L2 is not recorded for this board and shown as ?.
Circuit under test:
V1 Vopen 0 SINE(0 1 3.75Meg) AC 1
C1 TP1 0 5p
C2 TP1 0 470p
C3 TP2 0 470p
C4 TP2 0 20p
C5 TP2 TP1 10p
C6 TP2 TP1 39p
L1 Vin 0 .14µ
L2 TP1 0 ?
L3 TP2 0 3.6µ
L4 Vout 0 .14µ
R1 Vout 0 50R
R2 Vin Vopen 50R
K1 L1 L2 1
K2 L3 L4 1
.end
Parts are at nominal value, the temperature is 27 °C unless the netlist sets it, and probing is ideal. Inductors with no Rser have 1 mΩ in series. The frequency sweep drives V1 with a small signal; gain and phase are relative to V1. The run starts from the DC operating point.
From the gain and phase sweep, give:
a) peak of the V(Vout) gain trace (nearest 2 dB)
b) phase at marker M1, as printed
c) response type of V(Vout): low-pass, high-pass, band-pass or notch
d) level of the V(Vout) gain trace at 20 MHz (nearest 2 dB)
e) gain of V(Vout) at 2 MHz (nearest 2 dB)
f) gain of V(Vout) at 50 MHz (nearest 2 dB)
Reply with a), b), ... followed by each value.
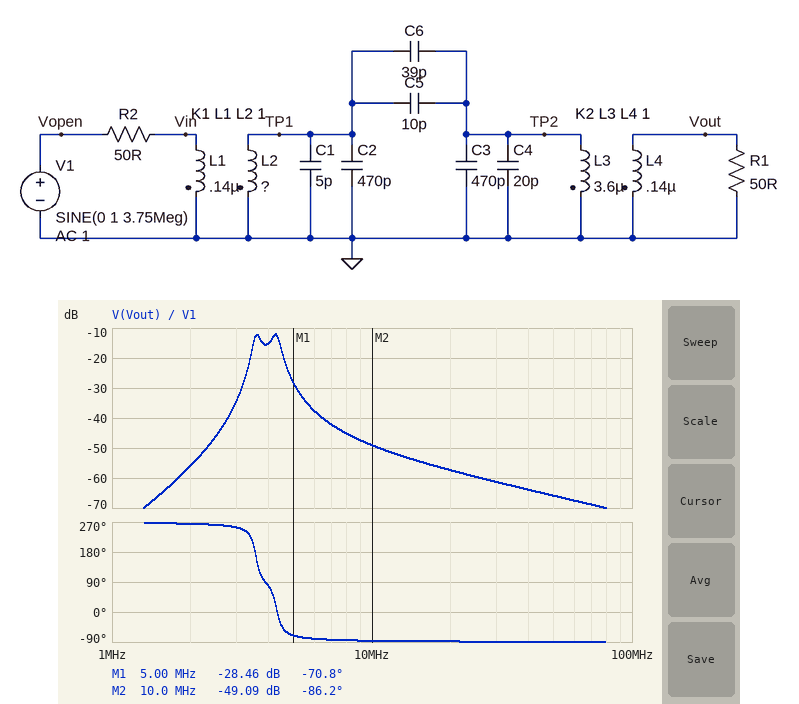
a) -12 dB
b) -70.8 deg
c) band-pass
d) -58 dB
e) -56 dB
f) -66 dB
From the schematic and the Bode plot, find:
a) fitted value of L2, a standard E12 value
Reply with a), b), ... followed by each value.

a) 2.7 µH
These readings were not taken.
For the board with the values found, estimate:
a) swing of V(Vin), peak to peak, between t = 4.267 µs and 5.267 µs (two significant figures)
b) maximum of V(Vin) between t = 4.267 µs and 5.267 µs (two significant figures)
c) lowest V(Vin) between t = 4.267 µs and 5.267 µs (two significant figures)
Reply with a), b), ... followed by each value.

a) 460 mV
b) 230 mV
c) -230 mV
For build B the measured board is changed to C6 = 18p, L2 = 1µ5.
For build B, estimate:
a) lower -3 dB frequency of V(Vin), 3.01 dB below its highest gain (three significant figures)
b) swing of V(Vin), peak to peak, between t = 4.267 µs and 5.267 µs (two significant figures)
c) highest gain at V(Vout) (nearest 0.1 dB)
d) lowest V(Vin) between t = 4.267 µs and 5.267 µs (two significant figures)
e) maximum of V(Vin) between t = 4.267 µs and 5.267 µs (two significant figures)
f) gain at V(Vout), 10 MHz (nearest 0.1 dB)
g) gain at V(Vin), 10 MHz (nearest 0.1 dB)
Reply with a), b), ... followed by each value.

a) 5.52 MHz
b) 220 mV
c) -24.7 dB
d) -110 mV
e) 110 mV
f) -48.9 dB
g) -21.0 dB
